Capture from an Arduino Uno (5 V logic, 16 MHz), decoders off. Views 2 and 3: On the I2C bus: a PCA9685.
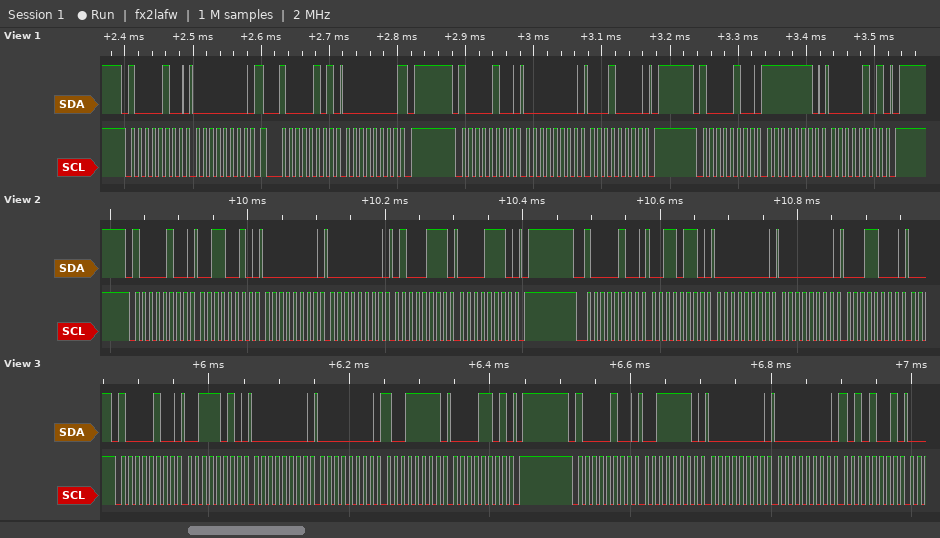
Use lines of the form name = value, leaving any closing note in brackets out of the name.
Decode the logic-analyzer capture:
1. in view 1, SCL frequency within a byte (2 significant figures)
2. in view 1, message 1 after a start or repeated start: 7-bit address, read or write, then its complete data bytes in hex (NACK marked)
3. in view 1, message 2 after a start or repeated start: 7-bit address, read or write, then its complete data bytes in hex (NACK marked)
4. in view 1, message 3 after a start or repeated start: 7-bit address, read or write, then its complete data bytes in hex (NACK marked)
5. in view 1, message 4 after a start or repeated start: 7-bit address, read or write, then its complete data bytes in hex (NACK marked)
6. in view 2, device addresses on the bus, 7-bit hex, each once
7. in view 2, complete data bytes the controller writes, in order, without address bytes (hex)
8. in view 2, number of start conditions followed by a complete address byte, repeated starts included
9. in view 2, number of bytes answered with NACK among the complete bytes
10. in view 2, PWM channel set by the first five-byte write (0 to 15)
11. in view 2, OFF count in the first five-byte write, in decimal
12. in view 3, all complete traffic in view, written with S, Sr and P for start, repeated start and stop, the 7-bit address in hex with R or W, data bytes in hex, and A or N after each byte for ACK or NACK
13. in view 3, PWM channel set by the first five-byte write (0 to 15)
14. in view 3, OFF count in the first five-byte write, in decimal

in view 1, SCL frequency within a byte = 100 kHz
in view 1, message 1 after a start or repeated start: 7-bit address, read or write, then its complete data bytes in hex = 0x42 write: 00
in view 1, message 2 after a start or repeated start: 7-bit address, read or write, then its complete data bytes in hex = 0x42 read: 00 NACK
in view 1, message 3 after a start or repeated start: 7-bit address, read or write, then its complete data bytes in hex = 0x42 write: 00 10
in view 1, message 4 after a start or repeated start: 7-bit address, read or write, then its complete data bytes in hex = 0x42 write: FE 05
in view 2, device addresses on the bus, 7-bit hex, each once = 0x42
in view 2, complete data bytes the controller writes, in order, without address bytes = 32 00 00 47 0E 36 00 00 18
in view 2, number of start conditions followed by a complete address byte, repeated starts included = 2
in view 2, number of bytes answered with NACK among the complete bytes = 0
in view 2, PWM channel set by the first five-byte write = 11
in view 2, OFF count in the first five-byte write, in decimal = 3655
in view 3, all complete traffic in view, written with S, Sr and P for start, repeated start and stop, the 7-bit address in hex with R or W, data bytes in hex, and A or N after each byte for ACK or NACK = S 42W A 3A A 00 A 00 A 9F A 0D A P S 42W A 3E A 00 A 00 A A9 A
in view 3, PWM channel set by the first five-byte write = 13
in view 3, OFF count in the first five-byte write, in decimal = 3487
